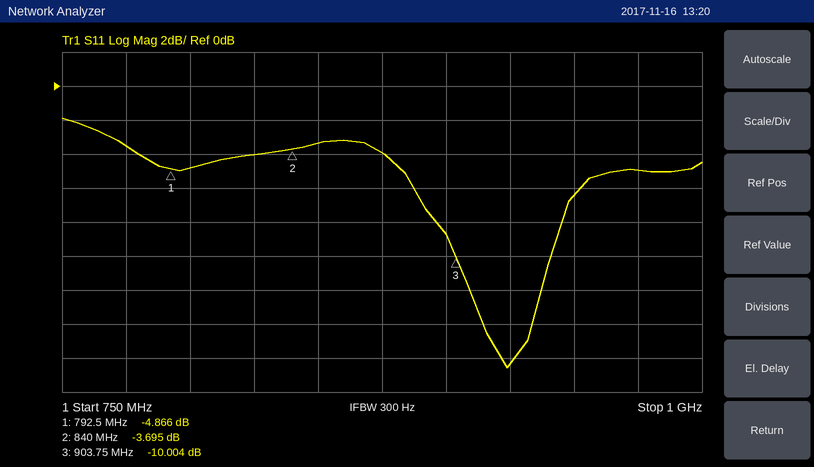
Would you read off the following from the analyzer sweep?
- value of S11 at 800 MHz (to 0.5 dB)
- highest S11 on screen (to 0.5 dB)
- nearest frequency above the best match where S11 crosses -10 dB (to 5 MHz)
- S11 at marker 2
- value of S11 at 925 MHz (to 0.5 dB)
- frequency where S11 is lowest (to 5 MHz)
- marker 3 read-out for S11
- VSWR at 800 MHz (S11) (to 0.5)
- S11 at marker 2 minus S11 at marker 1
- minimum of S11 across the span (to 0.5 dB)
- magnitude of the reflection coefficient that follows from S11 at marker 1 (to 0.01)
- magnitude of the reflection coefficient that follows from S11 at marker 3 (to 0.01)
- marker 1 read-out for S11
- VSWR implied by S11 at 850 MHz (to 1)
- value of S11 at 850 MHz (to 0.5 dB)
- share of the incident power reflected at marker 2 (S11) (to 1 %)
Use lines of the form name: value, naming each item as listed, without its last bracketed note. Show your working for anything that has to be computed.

value of S11 at 800 MHz: -5.0 dB
highest S11 on screen: -2.0 dB
nearest frequency above the best match where S11 crosses -10 dB: 940 MHz
S11 at marker 2: -3.695 dB
value of S11 at 925 MHz: -16.5 dB
frequency where S11 is lowest: 925 MHz
marker 3 read-out for S11: -10.004 dB
VSWR at 800 MHz (S11): |Γ| = 10^(-5/20) = 0.5623; VSWR = (1 + 0.5623)/(1 − 0.5623) ≈ 3.57, so 3.5 to the nearest 0.5
S11 at marker 2 minus S11 at marker 1: -3.695 − (-4.866) = 1.171 dB
minimum of S11 across the span: -16.5 dB
magnitude of the reflection coefficient that follows from S11 at marker 1: 10^(-4.866/20) ≈ 0.57
magnitude of the reflection coefficient that follows from S11 at marker 3: 10^(-10.004/20) ≈ 0.32
marker 1 read-out for S11: -4.866 dB
VSWR implied by S11 at 850 MHz: |Γ| = 10^(-3.5/20) = 0.6683; VSWR = (1 + 0.6683)/(1 − 0.6683) ≈ 5
value of S11 at 850 MHz: -3.5 dB
share of the incident power reflected at marker 2 (S11): 10^(-3.695/10) ≈ 43 %
